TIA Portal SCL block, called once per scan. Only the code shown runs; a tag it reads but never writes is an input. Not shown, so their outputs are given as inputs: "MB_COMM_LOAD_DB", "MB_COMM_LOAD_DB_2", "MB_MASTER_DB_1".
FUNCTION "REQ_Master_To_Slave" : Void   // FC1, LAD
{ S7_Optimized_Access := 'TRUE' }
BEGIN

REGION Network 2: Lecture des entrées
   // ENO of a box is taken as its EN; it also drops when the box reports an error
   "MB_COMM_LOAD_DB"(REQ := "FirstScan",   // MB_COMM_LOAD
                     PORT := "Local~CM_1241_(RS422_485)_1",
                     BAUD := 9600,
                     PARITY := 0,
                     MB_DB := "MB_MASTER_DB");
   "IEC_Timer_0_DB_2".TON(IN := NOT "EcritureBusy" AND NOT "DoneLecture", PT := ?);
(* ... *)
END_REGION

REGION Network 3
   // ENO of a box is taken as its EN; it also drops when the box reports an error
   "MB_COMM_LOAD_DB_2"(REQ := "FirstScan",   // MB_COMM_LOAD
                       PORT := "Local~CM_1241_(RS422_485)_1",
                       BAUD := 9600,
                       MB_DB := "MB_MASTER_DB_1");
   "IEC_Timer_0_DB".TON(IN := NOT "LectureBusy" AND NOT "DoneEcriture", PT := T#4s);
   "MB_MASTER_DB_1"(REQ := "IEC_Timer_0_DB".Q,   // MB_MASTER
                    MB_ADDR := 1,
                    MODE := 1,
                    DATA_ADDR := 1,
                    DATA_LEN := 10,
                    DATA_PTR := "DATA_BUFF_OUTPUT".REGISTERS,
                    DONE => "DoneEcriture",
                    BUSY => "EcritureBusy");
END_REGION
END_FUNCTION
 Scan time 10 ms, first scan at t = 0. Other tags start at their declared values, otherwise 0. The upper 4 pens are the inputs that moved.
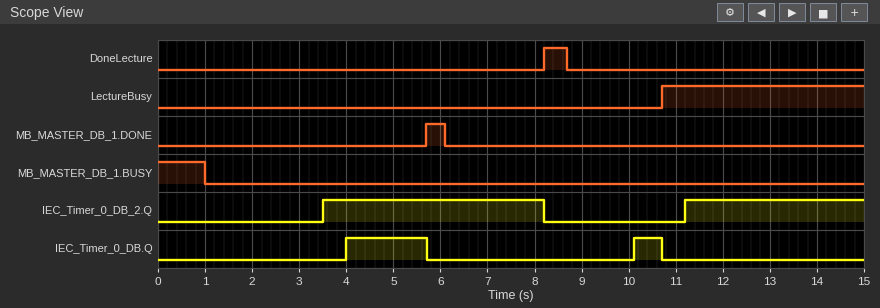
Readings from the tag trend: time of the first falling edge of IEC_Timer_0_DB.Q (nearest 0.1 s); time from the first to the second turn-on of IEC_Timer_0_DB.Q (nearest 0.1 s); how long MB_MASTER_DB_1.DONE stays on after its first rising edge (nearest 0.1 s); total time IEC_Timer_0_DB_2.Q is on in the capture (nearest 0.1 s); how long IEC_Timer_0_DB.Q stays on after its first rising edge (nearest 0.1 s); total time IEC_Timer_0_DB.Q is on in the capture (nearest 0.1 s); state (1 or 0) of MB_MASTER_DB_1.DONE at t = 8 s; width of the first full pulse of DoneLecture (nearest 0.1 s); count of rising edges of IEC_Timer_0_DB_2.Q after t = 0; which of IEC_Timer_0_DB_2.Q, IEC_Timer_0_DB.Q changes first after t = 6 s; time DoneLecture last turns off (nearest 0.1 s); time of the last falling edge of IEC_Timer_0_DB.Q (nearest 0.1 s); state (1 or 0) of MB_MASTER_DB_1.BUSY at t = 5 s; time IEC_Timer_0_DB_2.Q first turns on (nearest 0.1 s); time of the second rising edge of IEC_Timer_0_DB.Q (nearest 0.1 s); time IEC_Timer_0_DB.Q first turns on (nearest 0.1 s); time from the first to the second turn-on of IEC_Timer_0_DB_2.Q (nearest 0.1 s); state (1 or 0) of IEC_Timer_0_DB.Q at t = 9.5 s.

5.7 s
6.1 s
0.4 s
8.5 s
1.7 s
2.3 s
0
0.5 s
2
IEC_Timer_0_DB_2.Q
8.7 s
10.7 s
0
3.5 s
10.1 s
4.0 s
7.7 s
0
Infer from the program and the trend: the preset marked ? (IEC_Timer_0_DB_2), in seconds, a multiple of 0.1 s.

2.5 s
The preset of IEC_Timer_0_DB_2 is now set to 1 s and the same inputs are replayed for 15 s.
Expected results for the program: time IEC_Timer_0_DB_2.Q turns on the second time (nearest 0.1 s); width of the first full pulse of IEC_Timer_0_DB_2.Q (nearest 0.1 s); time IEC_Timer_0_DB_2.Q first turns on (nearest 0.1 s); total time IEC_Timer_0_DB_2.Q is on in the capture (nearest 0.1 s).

9.7 s
6.2 s
2.0 s
11.5 s
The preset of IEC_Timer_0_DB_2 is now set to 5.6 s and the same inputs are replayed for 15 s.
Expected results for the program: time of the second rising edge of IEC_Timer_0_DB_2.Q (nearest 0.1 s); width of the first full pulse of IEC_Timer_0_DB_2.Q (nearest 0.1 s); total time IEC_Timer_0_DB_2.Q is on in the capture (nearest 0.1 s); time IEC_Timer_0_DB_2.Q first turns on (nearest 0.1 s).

14.3 s
1.6 s
2.3 s
6.6 s
